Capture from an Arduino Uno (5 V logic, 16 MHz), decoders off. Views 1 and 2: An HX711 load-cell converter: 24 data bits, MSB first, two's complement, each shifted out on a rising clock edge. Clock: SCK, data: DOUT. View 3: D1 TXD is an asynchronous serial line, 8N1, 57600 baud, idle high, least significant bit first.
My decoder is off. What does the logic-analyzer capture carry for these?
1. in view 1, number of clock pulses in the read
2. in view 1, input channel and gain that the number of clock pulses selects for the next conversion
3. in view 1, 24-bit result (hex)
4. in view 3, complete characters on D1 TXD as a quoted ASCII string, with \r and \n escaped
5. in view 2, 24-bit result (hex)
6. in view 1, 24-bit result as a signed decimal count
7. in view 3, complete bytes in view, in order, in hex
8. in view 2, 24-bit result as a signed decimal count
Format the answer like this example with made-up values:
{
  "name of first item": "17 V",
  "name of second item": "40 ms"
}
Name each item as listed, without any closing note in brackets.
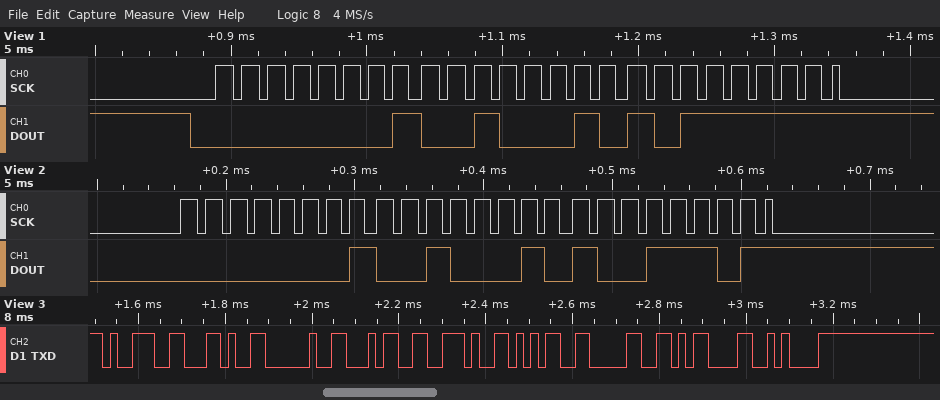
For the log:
{
  "in view 1, number of clock pulses in the read": "25",
  "in view 1, input channel and gain that the number of clock pulses selects for the next conversion": "channel A, gain 128",
  "in view 1, 24-bit result": "0x0122BF",
  "in view 3, complete characters on D1 TXD as a quoted ASCII string, with \\r and \\n escaped": "\"9, 4.50\\r\\n\"",
  "in view 2, 24-bit result": "0x01229D",
  "in view 1, 24-bit result as a signed decimal count": "74431",
  "in view 3, complete bytes in view, in order, in hex": "39 2C 20 34 2E 35 30 0D 0A",
  "in view 2, 24-bit result as a signed decimal count": "74397"
}
